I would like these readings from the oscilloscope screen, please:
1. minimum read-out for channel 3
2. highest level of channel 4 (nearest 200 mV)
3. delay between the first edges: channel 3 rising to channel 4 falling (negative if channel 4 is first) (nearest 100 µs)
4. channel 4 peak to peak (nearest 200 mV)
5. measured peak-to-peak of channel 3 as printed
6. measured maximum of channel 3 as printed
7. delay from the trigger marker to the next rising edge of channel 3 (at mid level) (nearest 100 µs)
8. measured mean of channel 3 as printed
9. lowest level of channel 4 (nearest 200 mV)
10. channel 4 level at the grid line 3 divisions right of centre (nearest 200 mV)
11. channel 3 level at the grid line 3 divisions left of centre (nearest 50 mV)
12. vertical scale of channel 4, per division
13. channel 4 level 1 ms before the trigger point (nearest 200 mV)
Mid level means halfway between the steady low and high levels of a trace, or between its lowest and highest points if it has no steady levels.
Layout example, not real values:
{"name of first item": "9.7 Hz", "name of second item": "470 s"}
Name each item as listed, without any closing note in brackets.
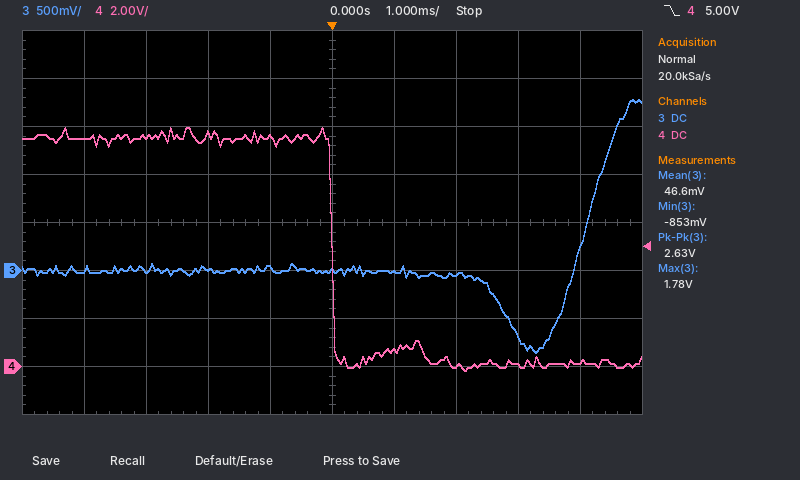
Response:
{"minimum read-out for channel 3": "-853 mV", "highest level of channel 4": "10.0 V", "delay between the first edges: channel 3 rising to channel 4 falling (negative if channel 4 is first)": "-4.1 ms", "channel 4 peak to peak": "10.2 V", "measured peak-to-peak of channel 3 as printed": "2.63 V", "measured maximum of channel 3 as printed": "1.78 V", "delay from the trigger marker to the next rising edge of channel 3 (at mid level)": "4.1 ms", "measured mean of channel 3 as printed": "46.6 mV", "lowest level of channel 4": "-200 mV", "channel 4 level at the grid line 3 divisions right of centre": "0.0 V", "channel 3 level at the grid line 3 divisions left of centre": "0 mV", "vertical scale of channel 4, per division": "2 V", "channel 4 level 1 ms before the trigger point": "9.6 V"}
